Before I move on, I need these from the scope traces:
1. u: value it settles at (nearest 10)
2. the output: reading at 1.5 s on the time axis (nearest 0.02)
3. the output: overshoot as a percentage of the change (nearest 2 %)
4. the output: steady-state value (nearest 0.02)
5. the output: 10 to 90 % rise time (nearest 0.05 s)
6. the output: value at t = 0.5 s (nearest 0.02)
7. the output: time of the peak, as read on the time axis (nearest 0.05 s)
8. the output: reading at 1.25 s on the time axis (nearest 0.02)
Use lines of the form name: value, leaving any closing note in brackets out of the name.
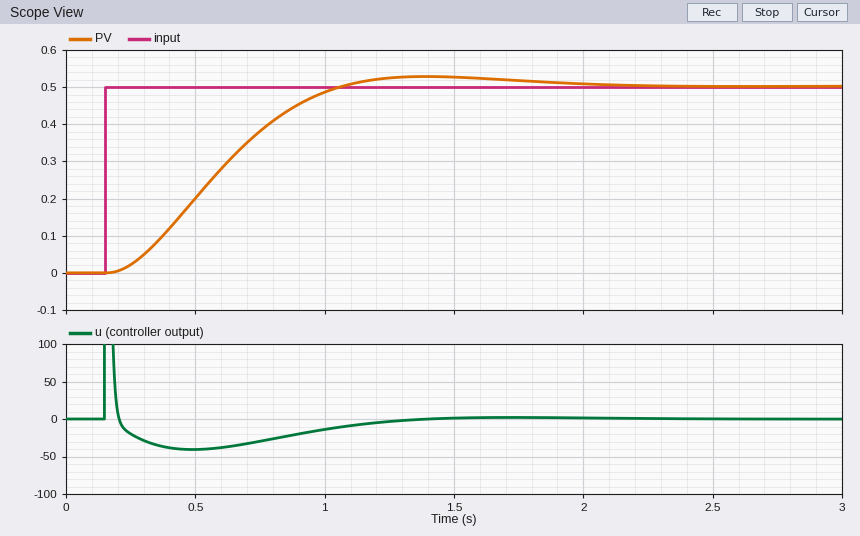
u: value it settles at: 0
the output: reading at 1.5 s on the time axis: 0.52
the output: overshoot as a percentage of the change: 6 %
the output: steady-state value: 0.50
the output: 10 to 90 % rise time: 0.60 s
the output: value at t = 0.5 s: 0.20
the output: time of the peak, as read on the time axis: 1.40 s
the output: reading at 1.25 s on the time axis: 0.52
